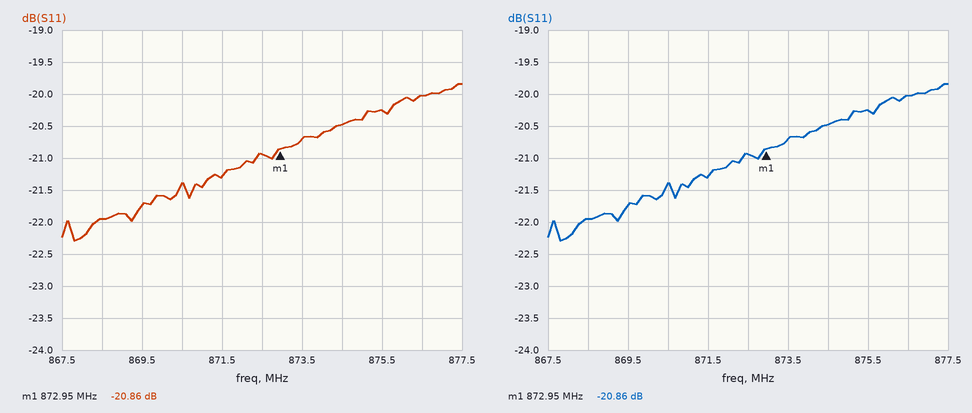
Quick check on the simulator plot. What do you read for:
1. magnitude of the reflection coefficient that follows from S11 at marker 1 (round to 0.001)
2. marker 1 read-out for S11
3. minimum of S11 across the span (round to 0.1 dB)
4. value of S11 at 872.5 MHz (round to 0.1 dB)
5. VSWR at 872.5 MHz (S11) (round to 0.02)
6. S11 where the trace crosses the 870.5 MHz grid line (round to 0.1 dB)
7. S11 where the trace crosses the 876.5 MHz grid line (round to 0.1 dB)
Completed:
0.091
-20.86 dB
-22.3 dB
-20.9 dB
1.20
-21.4 dB
-20.0 dB
